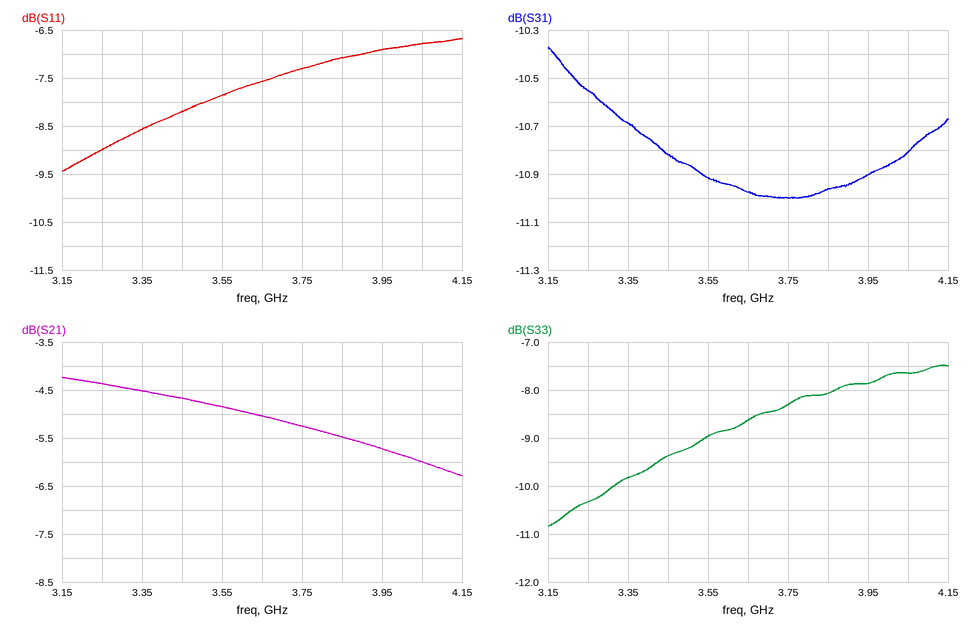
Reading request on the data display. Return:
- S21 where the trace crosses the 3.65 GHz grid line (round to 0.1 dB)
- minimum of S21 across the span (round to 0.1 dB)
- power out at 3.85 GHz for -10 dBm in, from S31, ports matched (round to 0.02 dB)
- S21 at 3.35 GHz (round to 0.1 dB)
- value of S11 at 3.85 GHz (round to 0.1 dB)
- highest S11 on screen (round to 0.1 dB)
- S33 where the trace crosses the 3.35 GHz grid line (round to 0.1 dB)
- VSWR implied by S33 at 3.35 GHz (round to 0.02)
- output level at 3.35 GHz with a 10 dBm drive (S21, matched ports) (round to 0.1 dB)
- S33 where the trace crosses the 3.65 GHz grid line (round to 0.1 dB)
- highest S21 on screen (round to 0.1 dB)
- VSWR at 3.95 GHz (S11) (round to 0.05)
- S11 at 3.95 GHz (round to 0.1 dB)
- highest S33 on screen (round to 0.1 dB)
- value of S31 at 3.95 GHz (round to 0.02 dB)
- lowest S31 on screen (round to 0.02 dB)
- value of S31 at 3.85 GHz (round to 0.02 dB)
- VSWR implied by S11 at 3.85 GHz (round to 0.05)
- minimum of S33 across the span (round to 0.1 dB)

-5.0 dB
-6.3 dB
-20.96 dBm
-4.5 dB
-7.1 dB
-6.7 dB
-9.8 dB
1.96
5.5 dBm
-8.6 dB
-4.2 dB
2.65
-6.9 dB
-7.5 dB
-10.90 dB
-11.00 dB
-10.96 dB
2.60
-10.8 dB
